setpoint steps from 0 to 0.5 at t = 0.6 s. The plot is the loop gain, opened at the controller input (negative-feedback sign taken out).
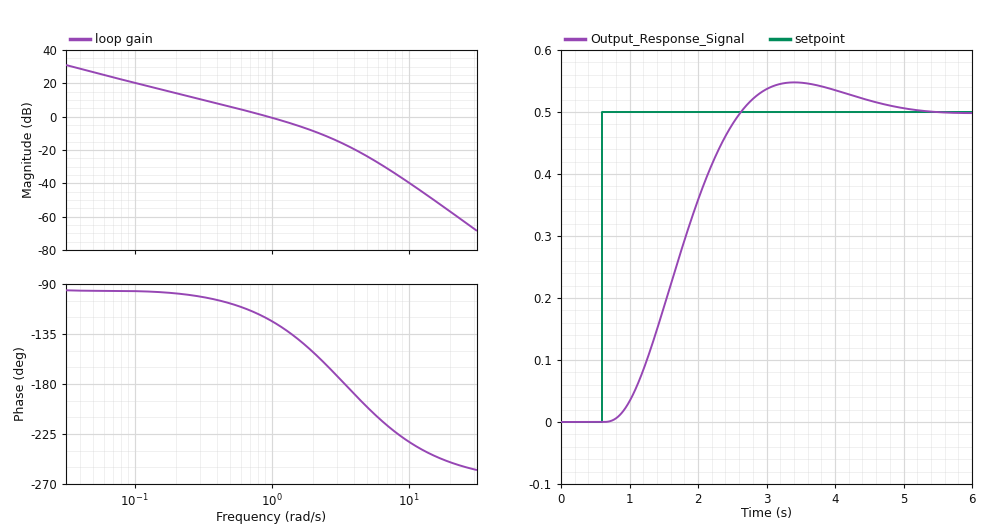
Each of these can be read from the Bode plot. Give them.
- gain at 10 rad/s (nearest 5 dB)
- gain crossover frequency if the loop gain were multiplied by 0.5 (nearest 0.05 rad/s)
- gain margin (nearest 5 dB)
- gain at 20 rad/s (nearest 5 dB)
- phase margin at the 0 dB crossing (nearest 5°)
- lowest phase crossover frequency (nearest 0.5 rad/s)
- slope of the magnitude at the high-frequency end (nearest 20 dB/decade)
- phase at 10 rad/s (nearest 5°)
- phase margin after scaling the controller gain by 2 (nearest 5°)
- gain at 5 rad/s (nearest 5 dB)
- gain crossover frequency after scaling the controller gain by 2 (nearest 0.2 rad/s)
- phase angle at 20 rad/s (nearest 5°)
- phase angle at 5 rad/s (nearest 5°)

-40 dB
0.50 rad/s
15 dB
-55 dB
60°
3.5 rad/s
-60 dB/decade
-230°
40°
-25 dB
1.6 rad/s
-250°
-200°
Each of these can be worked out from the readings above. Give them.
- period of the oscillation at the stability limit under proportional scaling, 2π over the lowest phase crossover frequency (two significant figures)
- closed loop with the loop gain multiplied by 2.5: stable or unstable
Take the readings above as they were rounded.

1.8 s
stable
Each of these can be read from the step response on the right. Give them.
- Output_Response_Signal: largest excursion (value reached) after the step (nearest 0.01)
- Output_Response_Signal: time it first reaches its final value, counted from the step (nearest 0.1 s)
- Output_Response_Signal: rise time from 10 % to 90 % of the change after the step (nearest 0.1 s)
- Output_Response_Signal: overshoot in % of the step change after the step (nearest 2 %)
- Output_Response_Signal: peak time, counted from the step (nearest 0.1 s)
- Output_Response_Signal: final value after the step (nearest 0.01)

0.55
2.0 s
1.3 s
10 %
2.8 s
0.50
